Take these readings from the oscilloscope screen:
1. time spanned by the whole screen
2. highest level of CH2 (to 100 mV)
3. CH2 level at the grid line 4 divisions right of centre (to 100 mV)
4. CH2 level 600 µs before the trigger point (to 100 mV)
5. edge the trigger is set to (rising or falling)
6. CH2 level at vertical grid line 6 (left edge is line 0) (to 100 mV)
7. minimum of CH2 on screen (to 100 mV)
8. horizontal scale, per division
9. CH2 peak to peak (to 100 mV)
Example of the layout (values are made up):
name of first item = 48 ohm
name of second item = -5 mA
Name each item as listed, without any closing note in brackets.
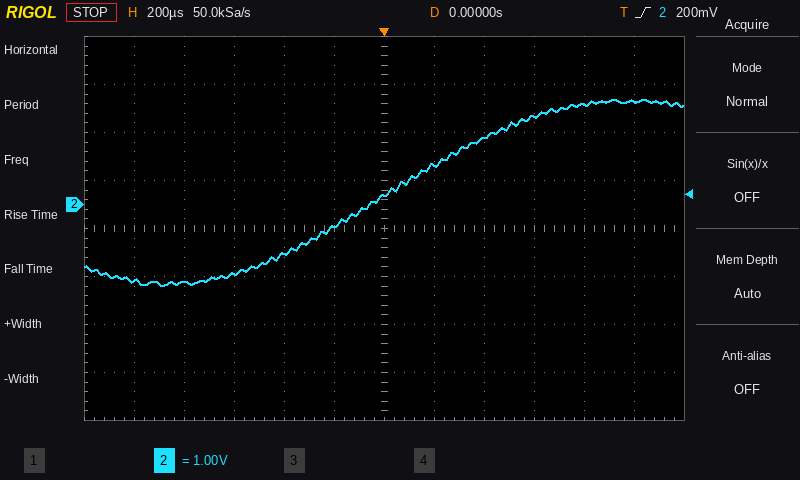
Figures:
time spanned by the whole screen = 2.4 ms
highest level of CH2 = 2.2 V
CH2 level at the grid line 4 divisions right of centre = 2.1 V
CH2 level 600 µs before the trigger point = -1.4 V
edge the trigger is set to = rising
CH2 level at vertical grid line 6 (left edge is line 0) = 200 mV
minimum of CH2 on screen = -1.7 V
horizontal scale, per division = 200 µs
CH2 peak to peak = 3.9 V
